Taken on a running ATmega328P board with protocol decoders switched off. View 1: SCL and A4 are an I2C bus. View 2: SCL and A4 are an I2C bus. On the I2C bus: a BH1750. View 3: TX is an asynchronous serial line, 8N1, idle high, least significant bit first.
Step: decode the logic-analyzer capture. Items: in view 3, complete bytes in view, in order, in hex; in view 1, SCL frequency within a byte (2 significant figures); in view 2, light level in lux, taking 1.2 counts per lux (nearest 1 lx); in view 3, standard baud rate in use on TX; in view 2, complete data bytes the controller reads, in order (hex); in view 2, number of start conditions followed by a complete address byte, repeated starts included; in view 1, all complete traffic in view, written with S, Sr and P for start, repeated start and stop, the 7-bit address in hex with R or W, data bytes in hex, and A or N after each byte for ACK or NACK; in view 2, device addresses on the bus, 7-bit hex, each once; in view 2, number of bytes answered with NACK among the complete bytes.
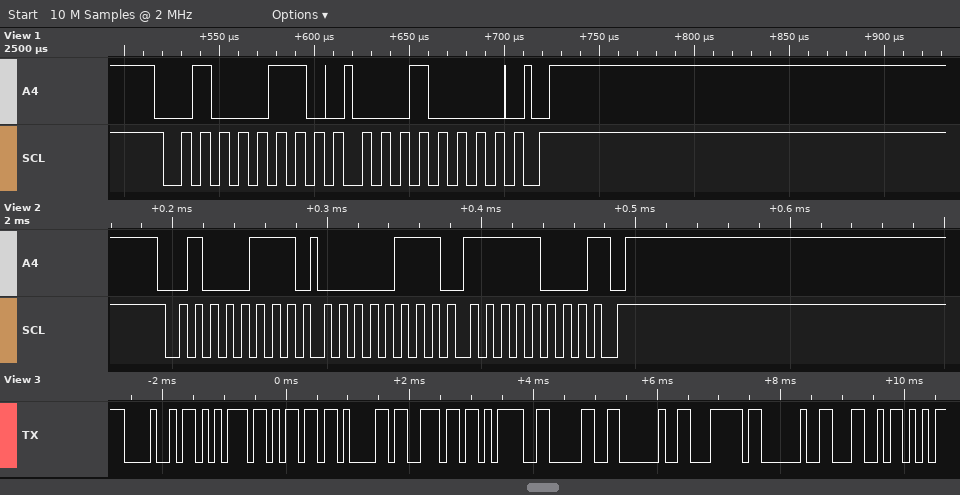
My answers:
48 75 6D 61 6E 3D 30 20 7C 20 4C
100 kHz
1700 lx
9600 baud
07 F8
1
S 23W A 10 A P
0x23
1
